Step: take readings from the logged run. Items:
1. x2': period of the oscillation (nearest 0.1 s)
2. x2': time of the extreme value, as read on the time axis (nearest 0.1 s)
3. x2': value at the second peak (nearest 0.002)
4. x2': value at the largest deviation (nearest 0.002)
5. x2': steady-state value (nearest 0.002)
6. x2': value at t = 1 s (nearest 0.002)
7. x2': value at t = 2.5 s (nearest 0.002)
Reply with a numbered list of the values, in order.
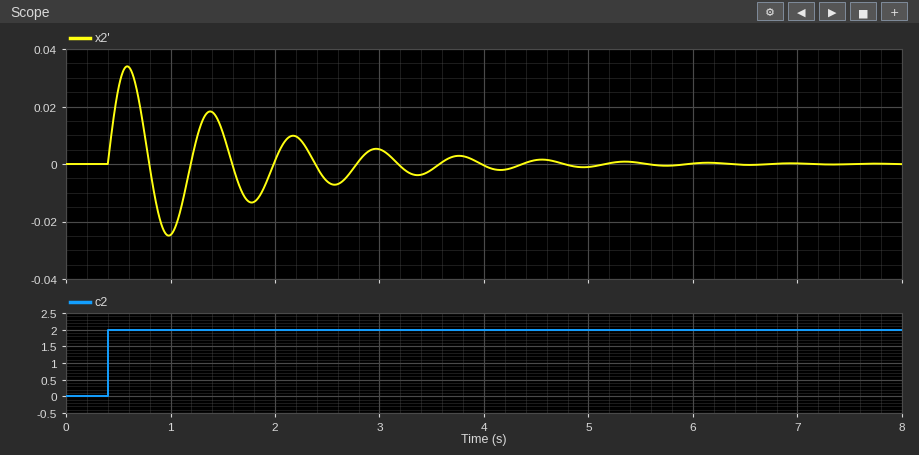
1. 0.8 s
2. 0.6 s
3. 0.018
4. 0.034
5. 0.000
6. -0.024
7. -0.006
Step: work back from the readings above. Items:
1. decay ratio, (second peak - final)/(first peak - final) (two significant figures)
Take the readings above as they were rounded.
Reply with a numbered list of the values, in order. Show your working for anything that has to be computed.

1. (0.018 - 0) / (0.034 - 0) = 0.53
